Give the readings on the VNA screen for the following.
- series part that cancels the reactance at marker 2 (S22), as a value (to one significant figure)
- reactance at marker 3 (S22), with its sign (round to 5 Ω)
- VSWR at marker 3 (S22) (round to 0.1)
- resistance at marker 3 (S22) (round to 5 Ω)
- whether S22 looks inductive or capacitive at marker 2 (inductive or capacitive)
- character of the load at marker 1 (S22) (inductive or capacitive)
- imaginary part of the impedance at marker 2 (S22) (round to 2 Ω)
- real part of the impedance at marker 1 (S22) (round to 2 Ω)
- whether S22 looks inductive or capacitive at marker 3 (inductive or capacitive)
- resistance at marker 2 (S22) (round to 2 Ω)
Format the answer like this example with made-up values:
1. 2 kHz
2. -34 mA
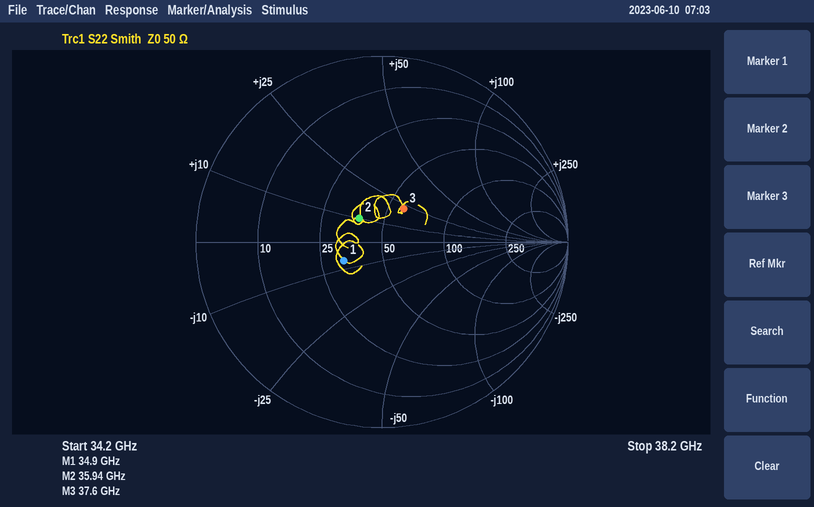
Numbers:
1. 400 fF
2. +20 Ω
3. 1.5
4. 60 Ω
5. inductive
6. capacitive
7. +10 Ω
8. 32 Ω
9. inductive
10. 38 Ω
